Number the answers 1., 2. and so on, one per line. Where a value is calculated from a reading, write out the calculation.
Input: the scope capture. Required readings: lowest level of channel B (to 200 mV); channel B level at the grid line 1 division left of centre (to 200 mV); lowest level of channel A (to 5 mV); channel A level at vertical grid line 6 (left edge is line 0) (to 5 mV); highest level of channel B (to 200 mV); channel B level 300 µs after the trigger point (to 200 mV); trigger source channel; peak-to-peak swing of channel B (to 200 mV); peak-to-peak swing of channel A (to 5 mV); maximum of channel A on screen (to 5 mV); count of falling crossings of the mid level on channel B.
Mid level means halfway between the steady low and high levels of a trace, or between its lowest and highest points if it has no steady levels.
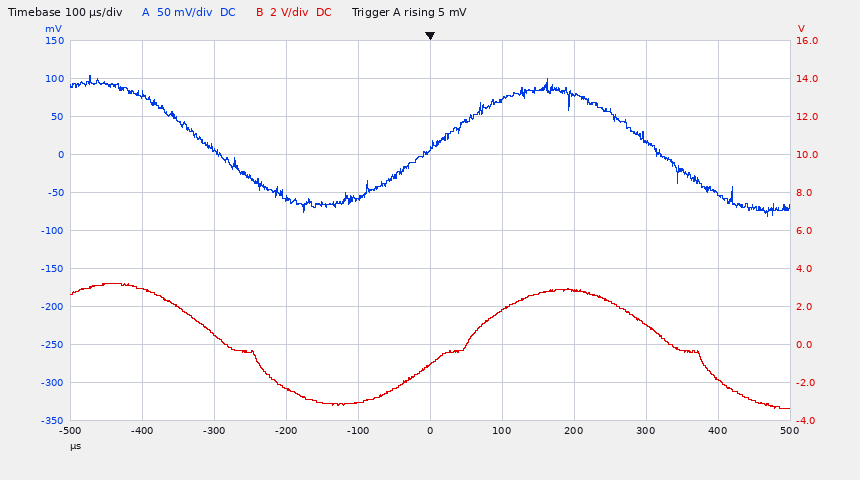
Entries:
1. -3.4 V
2. -3.0 V
3. -80 mV
4. 70 mV
5. 3.2 V
6. 1.0 V
7. channel A
8. 3.2 V − (-3.4 V) = 6.6 V
9. 105 mV − (-80 mV) = 185 mV
10. 105 mV
11. 2
